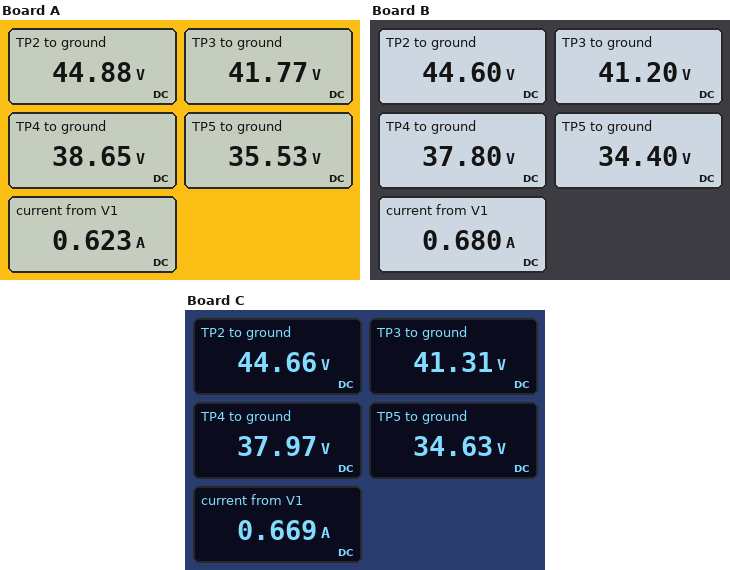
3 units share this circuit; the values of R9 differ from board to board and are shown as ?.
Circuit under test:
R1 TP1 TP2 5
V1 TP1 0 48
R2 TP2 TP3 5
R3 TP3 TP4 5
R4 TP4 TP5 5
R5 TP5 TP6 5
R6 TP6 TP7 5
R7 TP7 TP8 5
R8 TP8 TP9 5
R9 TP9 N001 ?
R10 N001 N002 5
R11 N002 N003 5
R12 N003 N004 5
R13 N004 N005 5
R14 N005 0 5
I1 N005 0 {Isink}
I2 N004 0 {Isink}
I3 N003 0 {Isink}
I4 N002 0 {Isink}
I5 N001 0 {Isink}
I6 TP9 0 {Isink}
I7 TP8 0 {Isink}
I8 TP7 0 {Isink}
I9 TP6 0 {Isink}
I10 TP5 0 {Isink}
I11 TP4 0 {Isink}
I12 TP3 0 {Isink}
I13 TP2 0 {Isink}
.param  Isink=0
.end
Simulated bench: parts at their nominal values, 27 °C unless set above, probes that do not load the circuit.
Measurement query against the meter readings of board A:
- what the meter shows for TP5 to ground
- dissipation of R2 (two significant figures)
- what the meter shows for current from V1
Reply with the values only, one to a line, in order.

35.53 V
1.9 W
0.623 A
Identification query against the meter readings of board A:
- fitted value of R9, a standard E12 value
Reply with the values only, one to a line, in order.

12 Ω
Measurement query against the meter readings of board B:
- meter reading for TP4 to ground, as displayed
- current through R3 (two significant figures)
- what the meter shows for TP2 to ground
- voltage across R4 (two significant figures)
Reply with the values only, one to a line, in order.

37.80 V
680 mA
44.60 V
3.4 V
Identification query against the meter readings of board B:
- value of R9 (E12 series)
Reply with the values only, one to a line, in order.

5.6 Ω
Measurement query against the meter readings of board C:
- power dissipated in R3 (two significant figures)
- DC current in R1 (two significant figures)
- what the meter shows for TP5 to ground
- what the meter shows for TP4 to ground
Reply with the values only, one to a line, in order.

2.2 W
670 mA
34.63 V
37.97 V
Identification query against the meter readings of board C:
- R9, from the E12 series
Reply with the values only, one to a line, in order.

6.8 Ω
